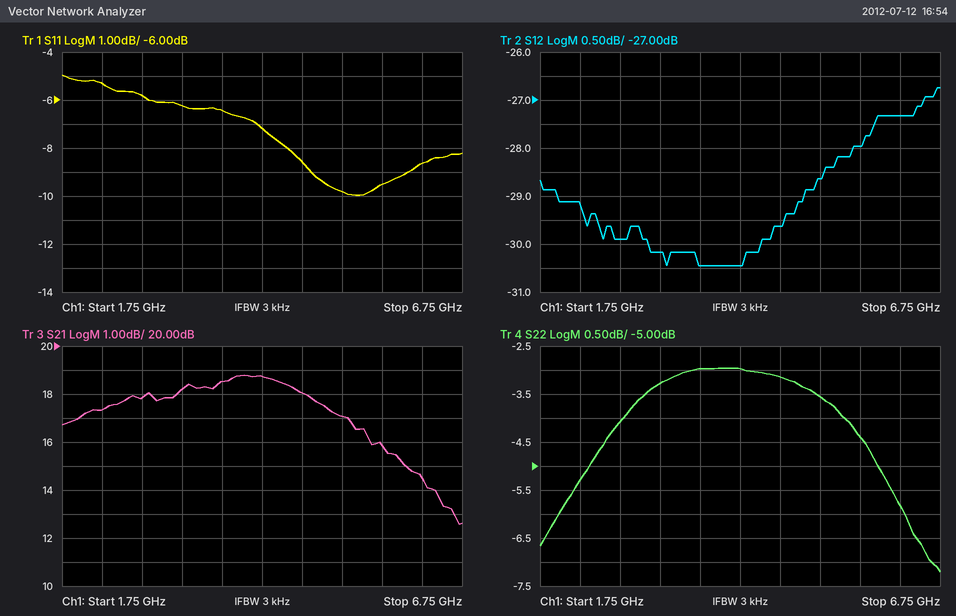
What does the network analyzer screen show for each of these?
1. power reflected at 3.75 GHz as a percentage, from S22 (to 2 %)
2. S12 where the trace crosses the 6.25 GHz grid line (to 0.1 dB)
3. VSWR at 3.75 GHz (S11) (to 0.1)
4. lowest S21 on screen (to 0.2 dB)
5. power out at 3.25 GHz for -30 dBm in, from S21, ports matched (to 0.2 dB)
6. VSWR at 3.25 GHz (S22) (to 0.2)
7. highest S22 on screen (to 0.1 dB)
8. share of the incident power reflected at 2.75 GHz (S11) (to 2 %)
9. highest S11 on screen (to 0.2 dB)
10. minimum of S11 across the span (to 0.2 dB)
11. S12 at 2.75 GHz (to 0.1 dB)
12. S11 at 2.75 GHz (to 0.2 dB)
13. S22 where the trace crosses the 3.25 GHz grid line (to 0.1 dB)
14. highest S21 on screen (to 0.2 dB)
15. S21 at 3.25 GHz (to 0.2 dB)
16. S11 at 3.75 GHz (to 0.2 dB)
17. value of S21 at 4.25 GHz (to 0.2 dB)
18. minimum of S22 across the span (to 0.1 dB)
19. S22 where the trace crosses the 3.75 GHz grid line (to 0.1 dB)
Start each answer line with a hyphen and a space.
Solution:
- 50 %
- -27.3 dB
- 2.8
- 12.6 dB
- -11.8 dBm
- 5.4
- -3.0 dB
- 26 %
- -5.0 dB
- -10.0 dB
- -29.9 dB
- -5.8 dB
- -3.3 dB
- 18.8 dB
- 18.2 dB
- -6.4 dB
- 18.8 dB
- -7.2 dB
- -3.0 dB
